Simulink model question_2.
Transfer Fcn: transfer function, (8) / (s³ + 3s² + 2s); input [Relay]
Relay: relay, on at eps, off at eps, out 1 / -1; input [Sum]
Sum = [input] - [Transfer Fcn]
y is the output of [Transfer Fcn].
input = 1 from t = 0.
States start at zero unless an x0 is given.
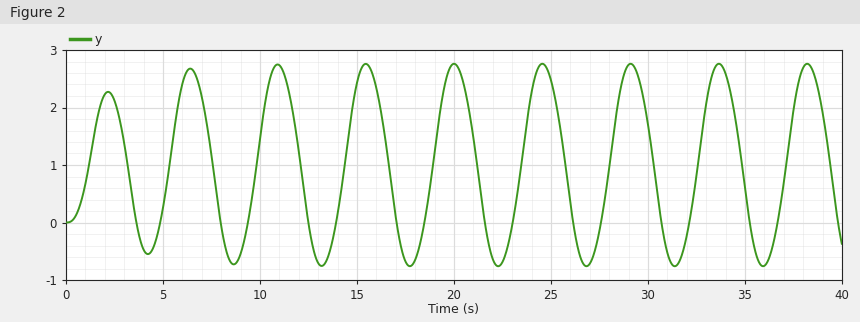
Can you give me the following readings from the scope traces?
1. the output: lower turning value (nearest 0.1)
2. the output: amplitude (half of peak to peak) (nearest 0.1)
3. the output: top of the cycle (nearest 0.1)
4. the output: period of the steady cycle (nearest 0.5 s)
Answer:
-0.8
1.8
2.8
4.5 s
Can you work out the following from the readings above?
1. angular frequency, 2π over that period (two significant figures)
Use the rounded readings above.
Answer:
1.4 rad/s
